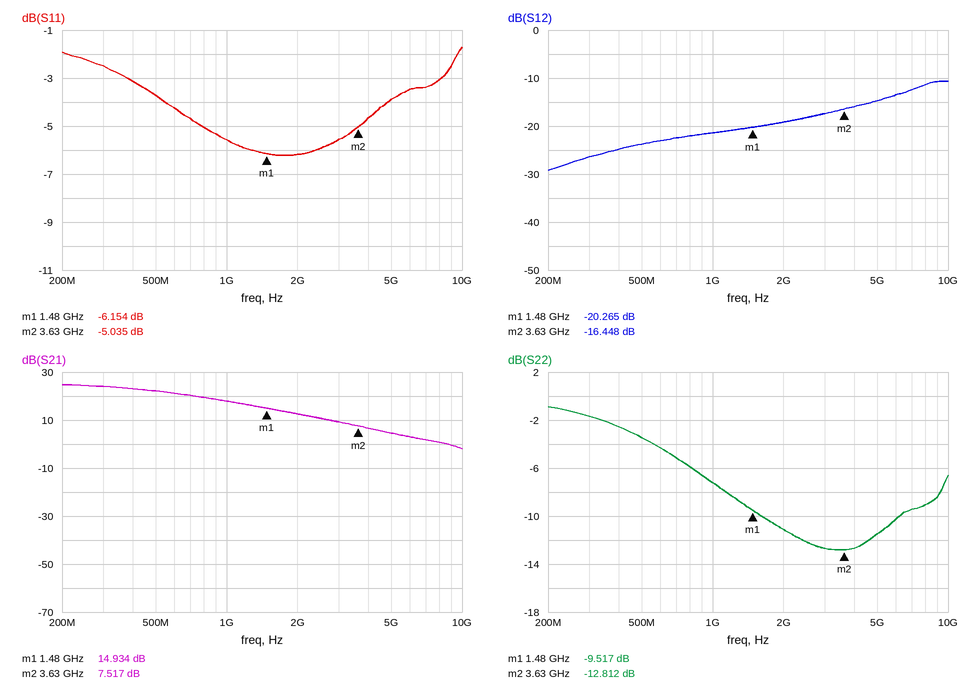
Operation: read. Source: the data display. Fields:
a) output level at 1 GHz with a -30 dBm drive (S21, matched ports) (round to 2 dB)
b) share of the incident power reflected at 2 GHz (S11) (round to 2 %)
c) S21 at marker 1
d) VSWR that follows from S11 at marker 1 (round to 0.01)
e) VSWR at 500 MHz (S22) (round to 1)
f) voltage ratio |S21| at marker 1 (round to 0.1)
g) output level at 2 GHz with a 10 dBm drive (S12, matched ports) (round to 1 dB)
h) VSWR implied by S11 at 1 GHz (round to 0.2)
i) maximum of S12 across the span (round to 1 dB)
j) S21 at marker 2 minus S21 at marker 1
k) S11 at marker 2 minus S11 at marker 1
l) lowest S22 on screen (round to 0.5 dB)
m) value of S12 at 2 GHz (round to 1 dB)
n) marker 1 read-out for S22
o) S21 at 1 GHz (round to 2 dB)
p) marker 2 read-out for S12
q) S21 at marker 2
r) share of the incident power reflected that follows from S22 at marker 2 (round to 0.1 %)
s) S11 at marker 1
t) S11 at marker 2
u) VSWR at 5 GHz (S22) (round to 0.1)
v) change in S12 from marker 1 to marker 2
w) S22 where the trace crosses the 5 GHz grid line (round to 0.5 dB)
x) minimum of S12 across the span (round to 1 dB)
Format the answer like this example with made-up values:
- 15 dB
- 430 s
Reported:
- -12 dBm
- 24 %
- 14.934 dB
- 2.94
- 5
- 5.6
- -9 dBm
- 3.2
- -11 dB
- -7.417 dB
- 1.119 dB
- -13.0 dB
- -19 dB
- -9.517 dB
- 18 dB
- -16.448 dB
- 7.517 dB
- 5.2 %
- -6.154 dB
- -5.035 dB
- 1.7
- 3.817 dB
- -11.5 dB
- -29 dB
